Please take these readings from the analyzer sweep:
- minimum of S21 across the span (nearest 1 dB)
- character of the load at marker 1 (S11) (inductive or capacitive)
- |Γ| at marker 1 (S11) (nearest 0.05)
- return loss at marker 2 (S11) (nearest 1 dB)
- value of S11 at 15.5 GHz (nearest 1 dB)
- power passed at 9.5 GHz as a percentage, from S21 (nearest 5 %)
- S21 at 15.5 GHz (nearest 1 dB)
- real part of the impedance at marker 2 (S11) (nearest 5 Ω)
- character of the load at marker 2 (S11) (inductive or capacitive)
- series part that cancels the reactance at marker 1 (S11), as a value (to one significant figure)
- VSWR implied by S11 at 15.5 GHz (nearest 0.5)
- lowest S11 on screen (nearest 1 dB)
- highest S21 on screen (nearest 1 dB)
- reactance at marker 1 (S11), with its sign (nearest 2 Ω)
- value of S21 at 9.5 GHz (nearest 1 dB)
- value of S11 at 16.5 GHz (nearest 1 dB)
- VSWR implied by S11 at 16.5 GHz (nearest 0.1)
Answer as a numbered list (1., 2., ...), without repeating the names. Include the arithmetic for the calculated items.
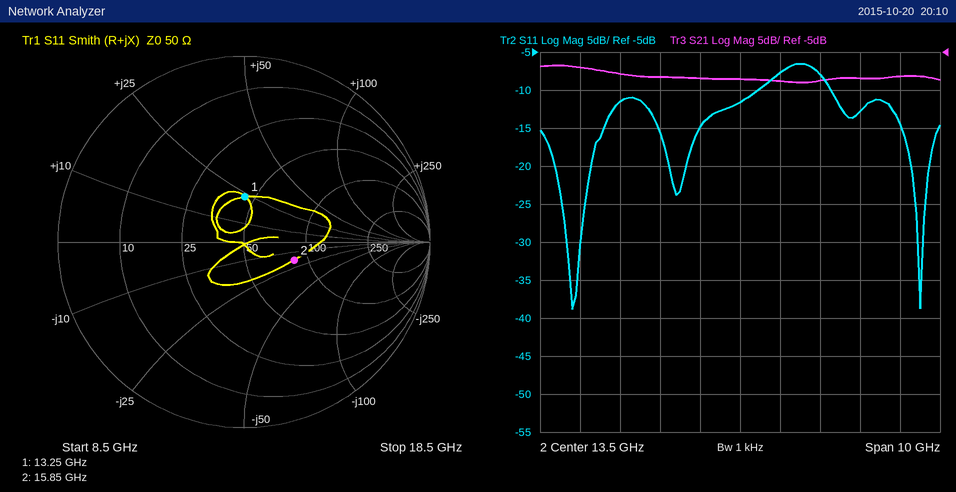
1. -9 dB
2. inductive
3. 0.25
4. 11 dB
5. -8 dB
6. 10^(-7/10) ≈ 20 %
7. -9 dB
8. 85 Ω
9. capacitive
10. C = 1/(2π × 13.25 GHz × 24 Ω) ≈ 500 fF
11. |Γ| = 10^(-8/20) = 0.3981; VSWR = (1 + 0.3981)/(1 − 0.3981) ≈ 2.32, so 2.5 to the nearest 0.5
12. -39 dB
13. -7 dB
14. +24 Ω
15. -7 dB
16. -13 dB
17. |Γ| = 10^(-13/20) = 0.2239; VSWR = (1 + 0.2239)/(1 − 0.2239) ≈ 1.6
